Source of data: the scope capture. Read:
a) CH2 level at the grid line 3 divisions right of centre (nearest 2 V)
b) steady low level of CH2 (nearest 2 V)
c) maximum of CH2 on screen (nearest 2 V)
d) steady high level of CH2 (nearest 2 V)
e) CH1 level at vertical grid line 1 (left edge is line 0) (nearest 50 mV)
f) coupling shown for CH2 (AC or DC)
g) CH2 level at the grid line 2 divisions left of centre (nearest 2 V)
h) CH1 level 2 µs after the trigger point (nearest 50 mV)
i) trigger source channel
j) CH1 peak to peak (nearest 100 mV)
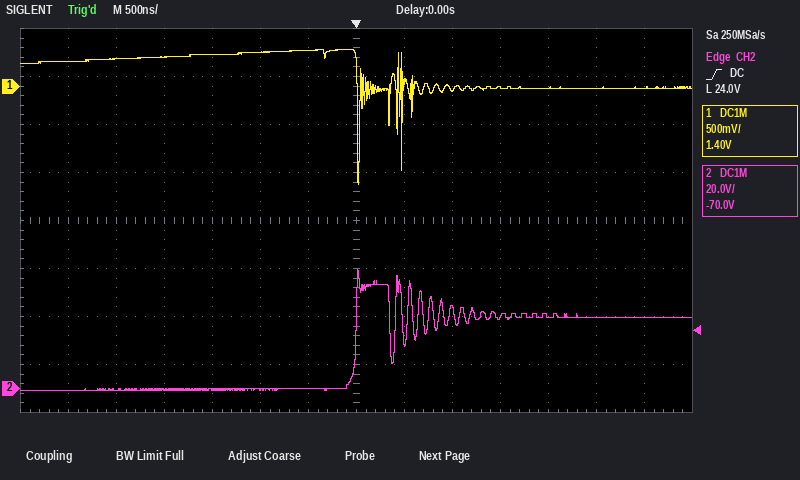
30 V
0 V
50 V
30 V
250 mV
DC
0 V
0 mV
CH2
1.40 V
